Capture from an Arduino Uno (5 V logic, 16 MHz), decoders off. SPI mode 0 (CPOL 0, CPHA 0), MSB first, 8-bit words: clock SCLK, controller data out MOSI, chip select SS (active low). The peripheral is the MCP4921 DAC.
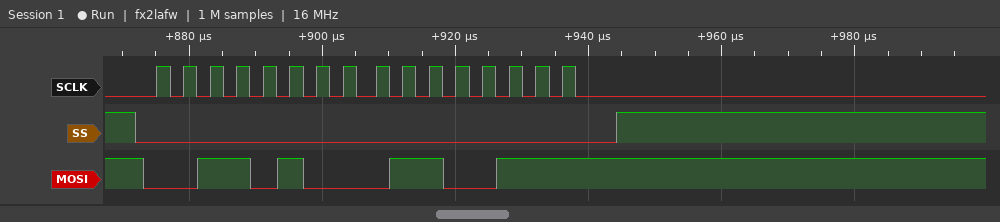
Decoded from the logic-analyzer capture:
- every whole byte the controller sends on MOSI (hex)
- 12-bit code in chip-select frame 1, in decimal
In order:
0x34 0x67
1127
